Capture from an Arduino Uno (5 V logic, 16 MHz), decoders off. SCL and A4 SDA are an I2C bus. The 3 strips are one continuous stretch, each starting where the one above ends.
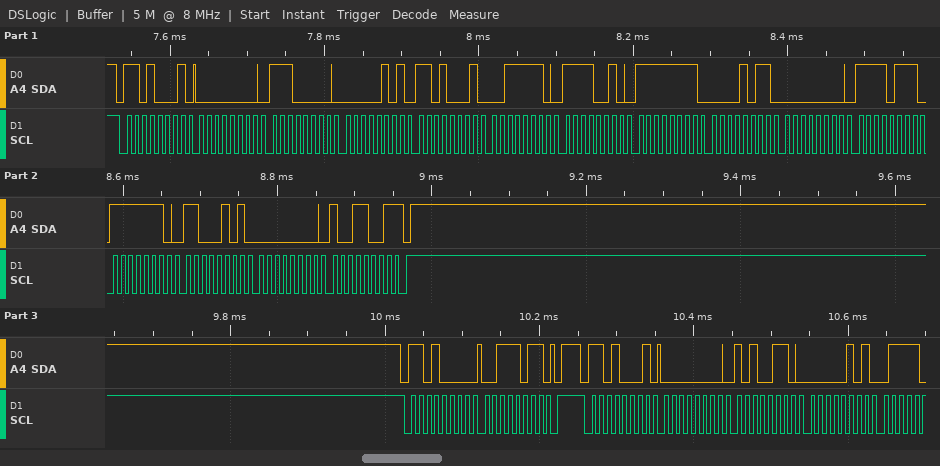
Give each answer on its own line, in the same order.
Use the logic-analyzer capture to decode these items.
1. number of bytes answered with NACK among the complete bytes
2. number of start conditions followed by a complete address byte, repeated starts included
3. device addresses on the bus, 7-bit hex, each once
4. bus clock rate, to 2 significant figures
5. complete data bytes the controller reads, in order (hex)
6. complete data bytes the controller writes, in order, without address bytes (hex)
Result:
1
3
0x68
100 kHz
00 E0 05 D1 3E F2 FF 0B 00 F7 FE C5 00 99 00 A6 05
3B
